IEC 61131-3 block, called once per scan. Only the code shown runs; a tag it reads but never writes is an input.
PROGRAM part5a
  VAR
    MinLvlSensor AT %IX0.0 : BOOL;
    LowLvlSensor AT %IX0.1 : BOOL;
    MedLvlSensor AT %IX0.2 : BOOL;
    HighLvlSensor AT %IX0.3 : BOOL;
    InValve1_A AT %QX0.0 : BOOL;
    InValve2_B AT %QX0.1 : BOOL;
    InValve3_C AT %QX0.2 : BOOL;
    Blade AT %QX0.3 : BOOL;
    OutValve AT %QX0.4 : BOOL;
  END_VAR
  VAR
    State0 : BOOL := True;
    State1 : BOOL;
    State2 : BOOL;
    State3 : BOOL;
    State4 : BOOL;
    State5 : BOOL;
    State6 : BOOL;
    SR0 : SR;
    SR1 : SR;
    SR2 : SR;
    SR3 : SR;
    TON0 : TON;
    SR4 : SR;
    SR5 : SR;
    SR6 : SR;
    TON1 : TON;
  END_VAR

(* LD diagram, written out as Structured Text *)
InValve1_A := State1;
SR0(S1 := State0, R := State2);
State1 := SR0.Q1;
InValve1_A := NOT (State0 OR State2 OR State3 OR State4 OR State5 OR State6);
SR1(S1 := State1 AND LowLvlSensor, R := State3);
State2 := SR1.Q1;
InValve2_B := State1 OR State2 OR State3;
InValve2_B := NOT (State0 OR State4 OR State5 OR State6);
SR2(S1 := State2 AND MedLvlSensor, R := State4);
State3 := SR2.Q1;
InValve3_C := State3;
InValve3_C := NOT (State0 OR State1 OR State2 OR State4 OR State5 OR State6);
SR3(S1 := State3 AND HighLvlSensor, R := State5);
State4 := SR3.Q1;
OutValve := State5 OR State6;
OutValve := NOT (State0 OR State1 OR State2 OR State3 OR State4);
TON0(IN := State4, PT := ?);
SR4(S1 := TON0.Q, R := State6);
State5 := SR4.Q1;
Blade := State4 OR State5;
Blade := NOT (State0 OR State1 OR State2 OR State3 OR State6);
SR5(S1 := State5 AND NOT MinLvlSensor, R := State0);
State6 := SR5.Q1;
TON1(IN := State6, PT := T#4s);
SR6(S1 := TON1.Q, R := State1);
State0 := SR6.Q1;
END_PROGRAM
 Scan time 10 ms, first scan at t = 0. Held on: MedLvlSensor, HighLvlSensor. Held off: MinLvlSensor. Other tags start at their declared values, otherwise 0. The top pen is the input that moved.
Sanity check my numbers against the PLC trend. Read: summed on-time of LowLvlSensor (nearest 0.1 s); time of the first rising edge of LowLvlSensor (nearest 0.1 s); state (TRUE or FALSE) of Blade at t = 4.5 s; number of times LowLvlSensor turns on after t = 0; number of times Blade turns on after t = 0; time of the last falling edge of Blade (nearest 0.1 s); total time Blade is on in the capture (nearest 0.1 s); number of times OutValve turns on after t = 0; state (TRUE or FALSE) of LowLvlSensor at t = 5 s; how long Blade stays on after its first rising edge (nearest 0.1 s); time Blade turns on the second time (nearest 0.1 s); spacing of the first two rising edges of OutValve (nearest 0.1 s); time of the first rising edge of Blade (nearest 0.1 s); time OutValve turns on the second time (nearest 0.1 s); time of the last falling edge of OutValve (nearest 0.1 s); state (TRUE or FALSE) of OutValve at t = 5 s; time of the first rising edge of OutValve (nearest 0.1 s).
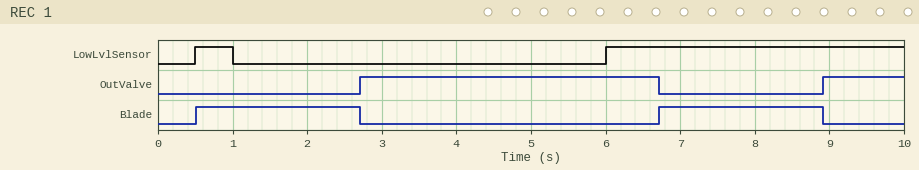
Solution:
4.5 s
0.5 s
FALSE
2
2
8.9 s
4.4 s
2
FALSE
2.2 s
6.7 s
6.2 s
0.5 s
8.9 s
6.7 s
TRUE
2.7 s
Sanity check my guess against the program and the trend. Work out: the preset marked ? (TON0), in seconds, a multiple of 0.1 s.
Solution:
2.2 s
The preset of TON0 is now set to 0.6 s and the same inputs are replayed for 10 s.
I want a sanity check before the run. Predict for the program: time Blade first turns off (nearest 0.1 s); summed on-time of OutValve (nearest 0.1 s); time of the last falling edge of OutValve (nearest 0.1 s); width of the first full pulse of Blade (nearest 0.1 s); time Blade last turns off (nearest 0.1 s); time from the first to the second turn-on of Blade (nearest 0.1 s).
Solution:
1.1 s
7.4 s
5.1 s
0.6 s
6.6 s
5.5 s
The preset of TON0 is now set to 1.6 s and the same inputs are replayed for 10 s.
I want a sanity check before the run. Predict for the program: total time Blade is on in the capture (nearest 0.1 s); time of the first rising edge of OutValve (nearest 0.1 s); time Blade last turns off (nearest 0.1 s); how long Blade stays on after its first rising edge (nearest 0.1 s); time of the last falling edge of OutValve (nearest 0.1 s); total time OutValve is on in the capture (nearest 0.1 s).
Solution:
3.2 s
2.1 s
7.7 s
1.6 s
6.1 s
6.3 s
